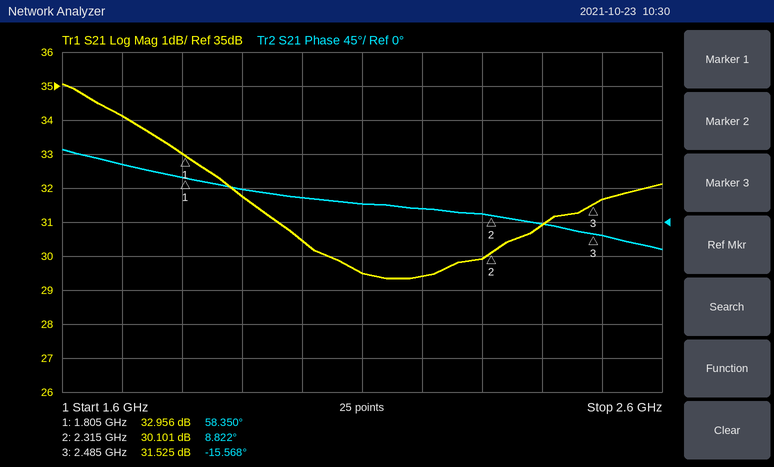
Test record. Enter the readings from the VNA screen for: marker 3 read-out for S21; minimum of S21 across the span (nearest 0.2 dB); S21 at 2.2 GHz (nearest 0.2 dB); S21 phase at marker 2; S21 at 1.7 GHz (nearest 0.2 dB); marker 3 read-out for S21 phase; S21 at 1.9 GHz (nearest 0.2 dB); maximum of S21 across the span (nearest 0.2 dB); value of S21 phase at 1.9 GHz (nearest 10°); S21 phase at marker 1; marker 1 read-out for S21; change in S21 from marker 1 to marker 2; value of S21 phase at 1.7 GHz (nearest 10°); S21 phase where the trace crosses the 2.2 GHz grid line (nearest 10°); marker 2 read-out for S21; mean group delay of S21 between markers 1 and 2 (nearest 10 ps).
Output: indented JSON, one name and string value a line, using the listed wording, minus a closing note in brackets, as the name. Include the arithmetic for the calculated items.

{
  "marker 3 read-out for S21": "31.525 dB",
  "minimum of S21 across the span": "29.4 dB",
  "S21 at 2.2 GHz": "29.4 dB",
  "S21 phase at marker 2": "8.822°",
  "S21 at 1.7 GHz": "34.2 dB",
  "marker 3 read-out for S21 phase": "-15.568°",
  "S21 at 1.9 GHz": "31.8 dB",
  "maximum of S21 across the span": "35.0 dB",
  "value of S21 phase at 1.9 GHz": "40°",
  "S21 phase at marker 1": "58.350°",
  "marker 1 read-out for S21": "32.956 dB",
  "change in S21 from marker 1 to marker 2": "30.101 − (32.956) = -2.855 dB",
  "value of S21 phase at 1.7 GHz": "80°",
  "S21 phase where the trace crosses the 2.2 GHz grid line": "20°",
  "marker 2 read-out for S21": "30.101 dB",
  "mean group delay of S21 between markers 1 and 2": "−(8.822° − (58.35°))/(360° × 510 MHz) ≈ 270 ps"
}
